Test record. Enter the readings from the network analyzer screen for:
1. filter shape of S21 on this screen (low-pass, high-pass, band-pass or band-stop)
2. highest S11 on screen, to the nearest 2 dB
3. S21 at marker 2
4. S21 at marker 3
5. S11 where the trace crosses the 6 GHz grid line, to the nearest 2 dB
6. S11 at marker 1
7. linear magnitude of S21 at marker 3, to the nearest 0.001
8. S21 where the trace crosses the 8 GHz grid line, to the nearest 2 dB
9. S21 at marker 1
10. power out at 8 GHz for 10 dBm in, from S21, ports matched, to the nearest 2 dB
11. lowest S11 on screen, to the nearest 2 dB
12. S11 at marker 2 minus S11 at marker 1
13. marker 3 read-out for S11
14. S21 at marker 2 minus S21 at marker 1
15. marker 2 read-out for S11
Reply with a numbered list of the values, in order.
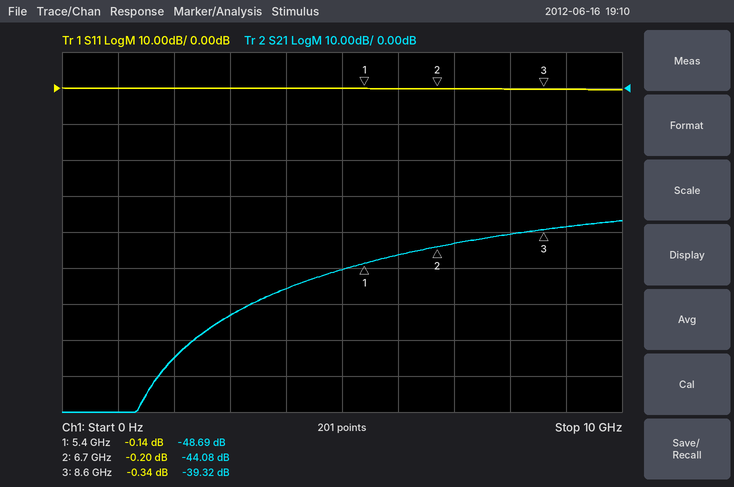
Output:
1. high-pass
2. 0 dB
3. -44.08 dB
4. -39.32 dB
5. 0 dB
6. -0.14 dB
7. 0.011
8. -40 dB
9. -48.69 dB
10. -30 dBm
11. 0 dB
12. -0.06 dB
13. -0.34 dB
14. 4.61 dB
15. -0.20 dB
